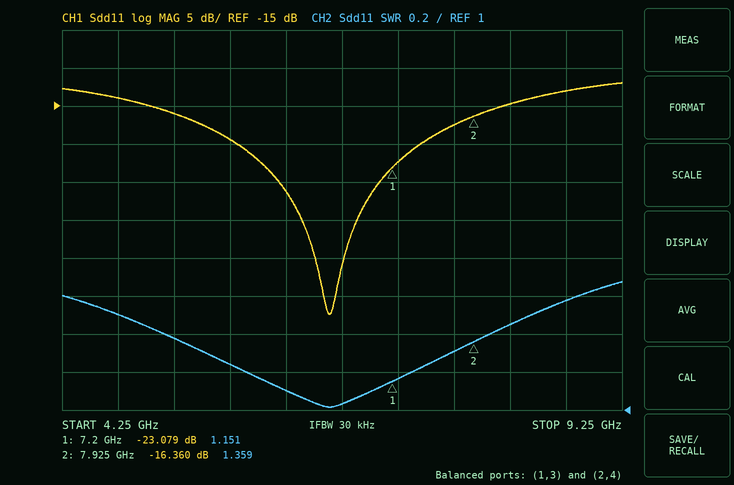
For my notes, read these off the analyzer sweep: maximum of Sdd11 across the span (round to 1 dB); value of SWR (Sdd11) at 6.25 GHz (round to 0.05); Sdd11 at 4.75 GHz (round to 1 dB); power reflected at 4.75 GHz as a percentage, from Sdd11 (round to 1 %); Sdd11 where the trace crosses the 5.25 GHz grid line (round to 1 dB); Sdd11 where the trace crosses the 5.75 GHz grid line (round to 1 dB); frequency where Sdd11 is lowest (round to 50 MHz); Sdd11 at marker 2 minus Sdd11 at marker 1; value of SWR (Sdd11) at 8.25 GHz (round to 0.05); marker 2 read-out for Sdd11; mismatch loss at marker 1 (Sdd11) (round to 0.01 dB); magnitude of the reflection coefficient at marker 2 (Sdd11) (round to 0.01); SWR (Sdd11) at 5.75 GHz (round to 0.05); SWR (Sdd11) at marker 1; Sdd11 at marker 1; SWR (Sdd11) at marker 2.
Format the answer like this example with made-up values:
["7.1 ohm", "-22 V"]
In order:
["-12 dB", "1.10", "-14 dB", "4 %", "-16 dB", "-19 dB", "6.65 GHz", "6.719 dB", "1.45", "-16.360 dB", "0.02 dB", "0.15", "1.25", "1.151", "-23.079 dB", "1.359"]
